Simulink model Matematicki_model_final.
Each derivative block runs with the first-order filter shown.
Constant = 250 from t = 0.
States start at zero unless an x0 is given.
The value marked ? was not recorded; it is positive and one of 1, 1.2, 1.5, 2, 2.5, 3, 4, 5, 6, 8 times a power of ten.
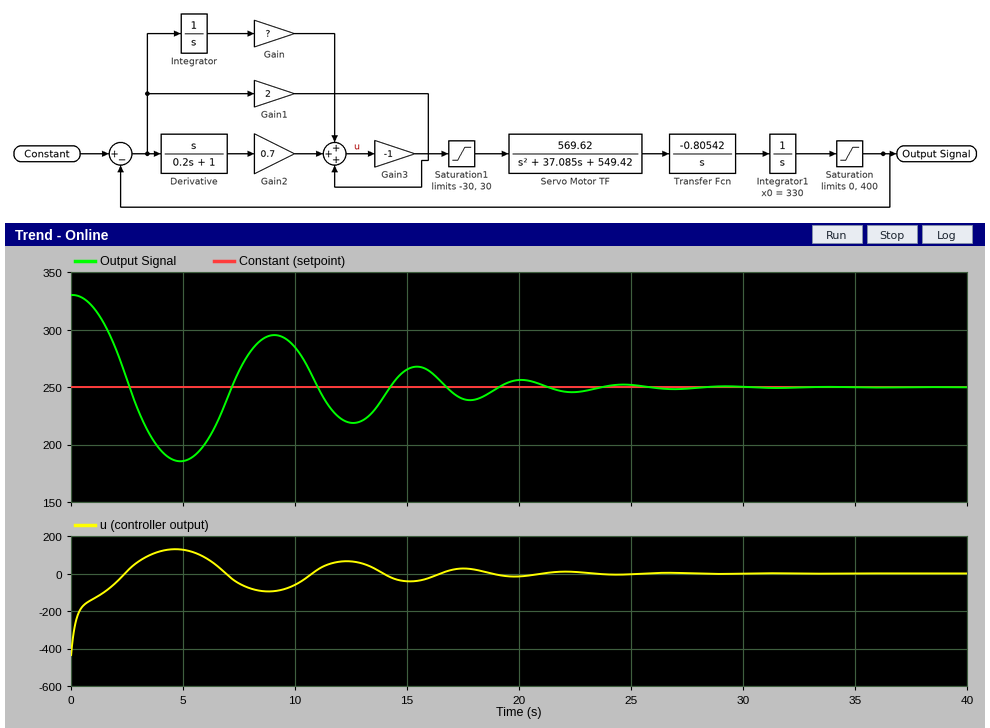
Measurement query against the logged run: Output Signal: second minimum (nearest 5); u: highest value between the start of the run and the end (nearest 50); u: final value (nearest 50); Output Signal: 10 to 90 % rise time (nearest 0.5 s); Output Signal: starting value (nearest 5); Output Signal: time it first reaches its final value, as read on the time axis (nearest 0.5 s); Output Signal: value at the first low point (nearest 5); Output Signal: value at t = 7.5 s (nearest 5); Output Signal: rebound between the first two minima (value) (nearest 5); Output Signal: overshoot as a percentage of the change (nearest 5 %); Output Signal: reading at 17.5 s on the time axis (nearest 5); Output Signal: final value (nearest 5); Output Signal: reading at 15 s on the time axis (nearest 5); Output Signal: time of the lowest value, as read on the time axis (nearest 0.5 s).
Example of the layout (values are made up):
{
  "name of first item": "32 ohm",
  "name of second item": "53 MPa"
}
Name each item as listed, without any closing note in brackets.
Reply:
{
  "Output Signal: second minimum": "220",
  "u: highest value between the start of the run and the end": "150",
  "u: final value": "0",
  "Output Signal: 10 to 90 % rise time": "1.5 s",
  "Output Signal: starting value": "330",
  "Output Signal: time it first reaches its final value, as read on the time axis": "2.5 s",
  "Output Signal: value at the first low point": "185",
  "Output Signal: value at t = 7.5 s": "265",
  "Output Signal: rebound between the first two minima (value)": "295",
  "Output Signal: overshoot as a percentage of the change": "80 %",
  "Output Signal: reading at 17.5 s on the time axis": "240",
  "Output Signal: final value": "250",
  "Output Signal: reading at 15 s on the time axis": "265",
  "Output Signal: time of the lowest value, as read on the time axis": "5.0 s"
}
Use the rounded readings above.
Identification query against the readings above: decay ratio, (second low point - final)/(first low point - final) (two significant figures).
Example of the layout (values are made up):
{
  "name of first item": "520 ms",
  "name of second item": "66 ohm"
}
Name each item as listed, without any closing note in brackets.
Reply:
{
  "decay ratio, (second low point - final)/(first low point - final)": "0.46"
}
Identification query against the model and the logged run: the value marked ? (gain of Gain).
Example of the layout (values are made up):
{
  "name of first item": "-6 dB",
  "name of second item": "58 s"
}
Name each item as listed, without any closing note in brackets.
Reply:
{
  "the value marked ?": "0.1"
}
